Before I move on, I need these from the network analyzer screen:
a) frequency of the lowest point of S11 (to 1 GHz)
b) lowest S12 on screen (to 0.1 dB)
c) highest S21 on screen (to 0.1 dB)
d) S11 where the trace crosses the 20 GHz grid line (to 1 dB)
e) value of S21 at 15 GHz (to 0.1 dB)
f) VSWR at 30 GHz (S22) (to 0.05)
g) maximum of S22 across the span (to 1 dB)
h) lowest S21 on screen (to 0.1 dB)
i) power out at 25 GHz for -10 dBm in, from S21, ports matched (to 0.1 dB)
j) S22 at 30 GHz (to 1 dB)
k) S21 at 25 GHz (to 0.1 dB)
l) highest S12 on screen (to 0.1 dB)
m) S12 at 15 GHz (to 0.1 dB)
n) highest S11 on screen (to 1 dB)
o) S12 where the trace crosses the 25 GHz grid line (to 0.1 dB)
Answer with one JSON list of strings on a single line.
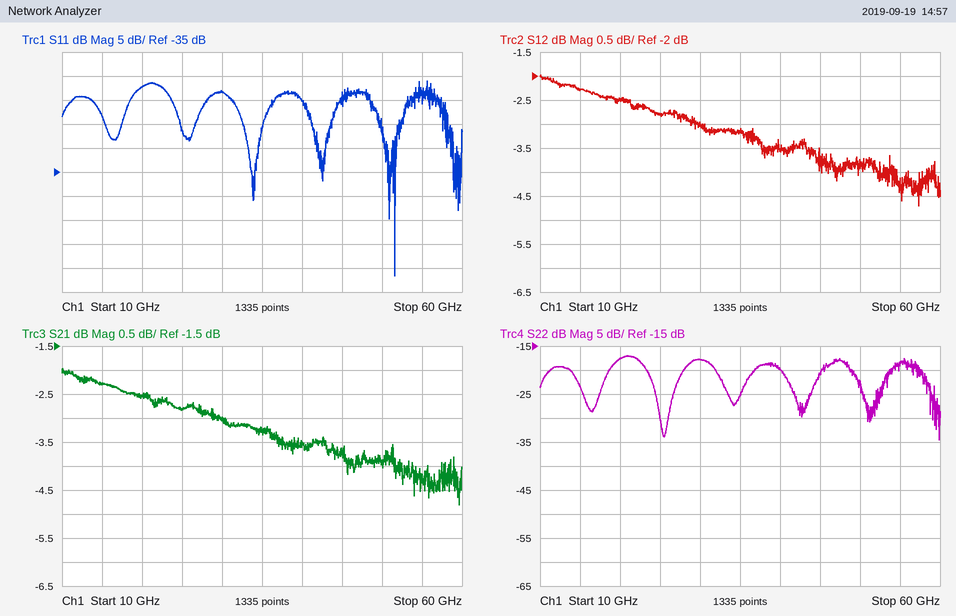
["52 GHz", "-4.7 dB", "-2.0 dB", "-17 dB", "-2.3 dB", "1.30", "-17 dB", "-4.8 dB", "-12.8 dBm", "-18 dB", "-2.8 dB", "-2.0 dB", "-2.3 dB", "-16 dB", "-2.8 dB"]
